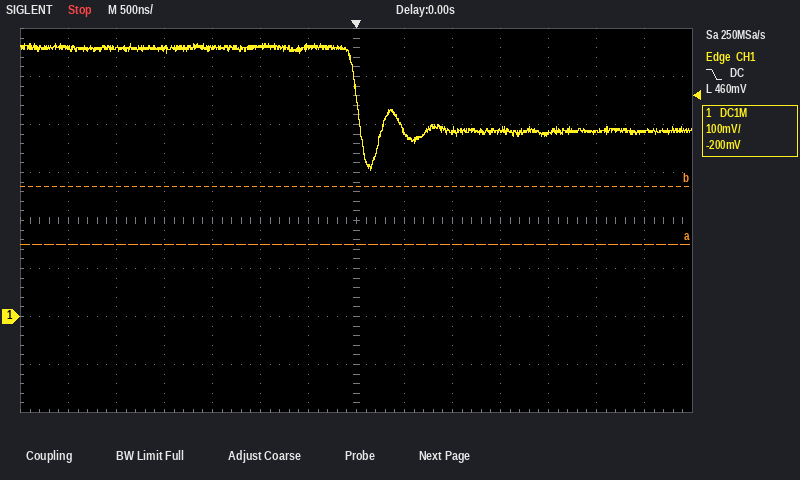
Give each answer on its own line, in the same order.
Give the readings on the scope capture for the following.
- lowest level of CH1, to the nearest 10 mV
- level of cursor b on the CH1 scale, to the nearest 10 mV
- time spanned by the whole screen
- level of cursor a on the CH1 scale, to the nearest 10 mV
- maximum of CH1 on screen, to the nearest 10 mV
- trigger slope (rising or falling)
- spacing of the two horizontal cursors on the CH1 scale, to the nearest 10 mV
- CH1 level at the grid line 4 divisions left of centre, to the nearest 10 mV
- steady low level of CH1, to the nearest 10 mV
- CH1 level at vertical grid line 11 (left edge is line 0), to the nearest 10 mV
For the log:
300 mV
270 mV
7 µs
150 mV
570 mV
falling
120 mV
560 mV
390 mV
380 mV
